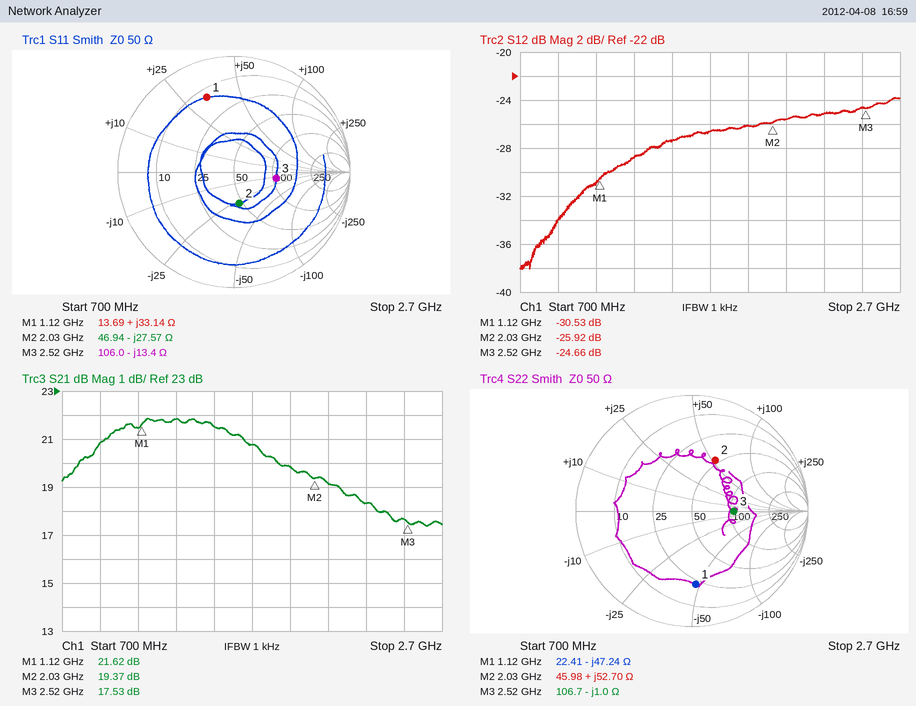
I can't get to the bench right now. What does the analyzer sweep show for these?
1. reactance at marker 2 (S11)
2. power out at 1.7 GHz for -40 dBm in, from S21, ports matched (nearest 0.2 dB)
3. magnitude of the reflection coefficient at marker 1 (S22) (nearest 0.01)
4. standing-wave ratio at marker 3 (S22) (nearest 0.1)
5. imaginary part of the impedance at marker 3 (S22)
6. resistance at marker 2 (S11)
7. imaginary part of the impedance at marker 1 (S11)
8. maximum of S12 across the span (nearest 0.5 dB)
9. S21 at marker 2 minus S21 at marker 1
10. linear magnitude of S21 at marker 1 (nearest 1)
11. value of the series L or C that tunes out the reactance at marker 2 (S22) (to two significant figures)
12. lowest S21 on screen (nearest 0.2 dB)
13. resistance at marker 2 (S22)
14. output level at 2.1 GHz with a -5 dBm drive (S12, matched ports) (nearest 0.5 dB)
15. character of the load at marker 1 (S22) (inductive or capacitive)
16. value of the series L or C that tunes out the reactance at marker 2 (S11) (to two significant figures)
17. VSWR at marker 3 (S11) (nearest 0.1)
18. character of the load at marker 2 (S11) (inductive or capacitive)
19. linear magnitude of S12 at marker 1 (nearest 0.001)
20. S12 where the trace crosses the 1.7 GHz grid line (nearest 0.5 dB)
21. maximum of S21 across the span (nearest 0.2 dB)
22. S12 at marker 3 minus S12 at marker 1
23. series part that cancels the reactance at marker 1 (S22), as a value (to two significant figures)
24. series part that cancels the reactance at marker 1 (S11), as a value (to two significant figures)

-27.57 Ω
-19.2 dBm
0.63
2.1
-1.0 Ω
46.94 Ω
+33.14 Ω
-24.0 dB
-2.25 dB
12
1.5 pF
17.4 dB
45.98 Ω
-30.5 dBm
capacitive
2.2 nH
2.2
capacitive
0.030
-26.5 dB
21.8 dB
5.87 dB
6.7 nH
4.3 pF
